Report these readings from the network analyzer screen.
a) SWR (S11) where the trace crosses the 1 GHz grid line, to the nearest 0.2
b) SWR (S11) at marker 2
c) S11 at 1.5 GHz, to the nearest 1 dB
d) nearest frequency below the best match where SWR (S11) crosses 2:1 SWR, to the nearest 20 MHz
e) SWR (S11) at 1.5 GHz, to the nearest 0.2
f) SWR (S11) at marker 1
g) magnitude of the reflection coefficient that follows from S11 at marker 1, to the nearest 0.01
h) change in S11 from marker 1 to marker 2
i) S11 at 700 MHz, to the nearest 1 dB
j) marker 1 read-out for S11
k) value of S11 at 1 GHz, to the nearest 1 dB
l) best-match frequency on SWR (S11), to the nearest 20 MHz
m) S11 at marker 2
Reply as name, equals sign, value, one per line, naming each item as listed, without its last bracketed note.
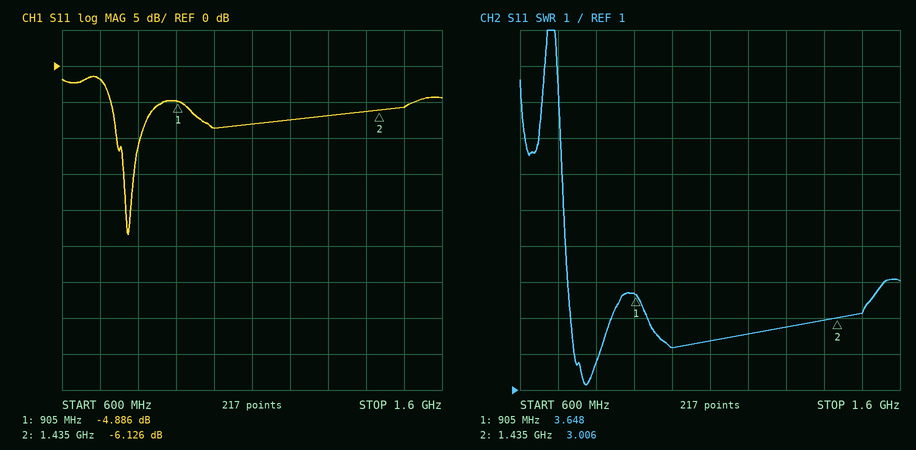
SWR (S11) where the trace crosses the 1 GHz grid line, to the nearest 0.2 = 2.2
SWR (S11) at marker 2 = 3.006
S11 at 1.5 GHz, to the nearest 1 dB = -6 dB
nearest frequency below the best match where SWR (S11) crosses 2:1 SWR, to the nearest 20 MHz = 740 MHz
SWR (S11) at 1.5 GHz, to the nearest 0.2 = 3.2
SWR (S11) at marker 1 = 3.648
magnitude of the reflection coefficient that follows from S11 at marker 1, to the nearest 0.01 = 0.57
change in S11 from marker 1 to marker 2 = -1.240 dB
S11 at 700 MHz, to the nearest 1 dB = -2 dB
marker 1 read-out for S11 = -4.886 dB
value of S11 at 1 GHz, to the nearest 1 dB = -9 dB
best-match frequency on SWR (S11), to the nearest 20 MHz = 780 MHz
S11 at marker 2 = -6.126 dB
